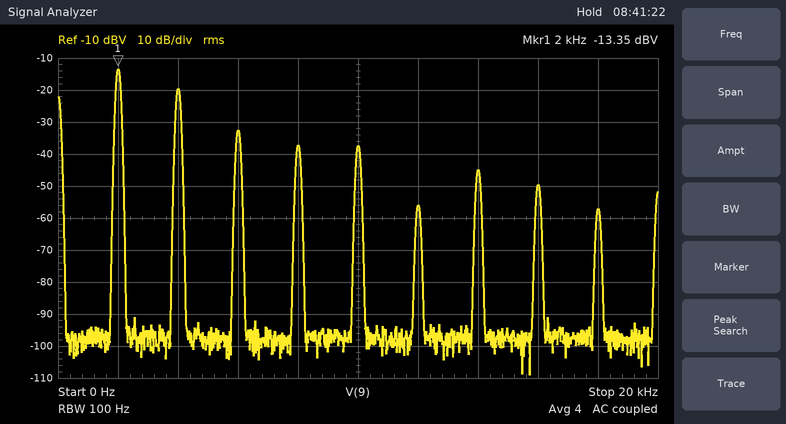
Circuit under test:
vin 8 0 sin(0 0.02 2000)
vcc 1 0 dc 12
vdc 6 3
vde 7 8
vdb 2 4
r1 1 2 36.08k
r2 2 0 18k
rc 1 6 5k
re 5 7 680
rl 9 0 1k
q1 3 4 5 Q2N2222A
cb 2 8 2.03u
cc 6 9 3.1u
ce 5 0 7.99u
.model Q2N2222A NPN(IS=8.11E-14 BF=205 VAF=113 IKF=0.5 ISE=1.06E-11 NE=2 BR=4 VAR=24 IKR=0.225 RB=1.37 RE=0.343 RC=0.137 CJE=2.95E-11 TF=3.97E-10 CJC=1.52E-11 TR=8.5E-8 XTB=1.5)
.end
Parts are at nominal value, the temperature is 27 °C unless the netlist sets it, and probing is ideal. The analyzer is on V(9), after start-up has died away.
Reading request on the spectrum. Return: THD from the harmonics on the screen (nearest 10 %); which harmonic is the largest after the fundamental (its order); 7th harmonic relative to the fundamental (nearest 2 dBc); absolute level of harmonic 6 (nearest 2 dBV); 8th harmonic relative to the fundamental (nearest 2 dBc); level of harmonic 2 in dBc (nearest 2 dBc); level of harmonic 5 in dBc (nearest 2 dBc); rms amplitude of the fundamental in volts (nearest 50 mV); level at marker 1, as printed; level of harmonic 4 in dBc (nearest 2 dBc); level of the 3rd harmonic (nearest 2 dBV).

50 %
2
-32 dBc
-56 dBV
-36 dBc
-6 dBc
-24 dBc
200 mV
-13.35 dBV
-24 dBc
-32 dBV
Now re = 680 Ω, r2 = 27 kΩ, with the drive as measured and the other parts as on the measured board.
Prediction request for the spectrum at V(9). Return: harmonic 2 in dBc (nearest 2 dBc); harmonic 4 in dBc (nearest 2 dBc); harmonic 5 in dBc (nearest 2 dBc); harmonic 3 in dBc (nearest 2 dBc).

-4 dBc
-28 dBc
-26 dBc
-12 dBc
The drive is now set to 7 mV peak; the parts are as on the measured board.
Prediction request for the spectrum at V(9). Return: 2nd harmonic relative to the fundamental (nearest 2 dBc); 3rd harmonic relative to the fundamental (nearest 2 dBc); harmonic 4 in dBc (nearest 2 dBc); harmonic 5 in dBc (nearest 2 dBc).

-14 dBc
-28 dBc
-40 dBc
-52 dBc
